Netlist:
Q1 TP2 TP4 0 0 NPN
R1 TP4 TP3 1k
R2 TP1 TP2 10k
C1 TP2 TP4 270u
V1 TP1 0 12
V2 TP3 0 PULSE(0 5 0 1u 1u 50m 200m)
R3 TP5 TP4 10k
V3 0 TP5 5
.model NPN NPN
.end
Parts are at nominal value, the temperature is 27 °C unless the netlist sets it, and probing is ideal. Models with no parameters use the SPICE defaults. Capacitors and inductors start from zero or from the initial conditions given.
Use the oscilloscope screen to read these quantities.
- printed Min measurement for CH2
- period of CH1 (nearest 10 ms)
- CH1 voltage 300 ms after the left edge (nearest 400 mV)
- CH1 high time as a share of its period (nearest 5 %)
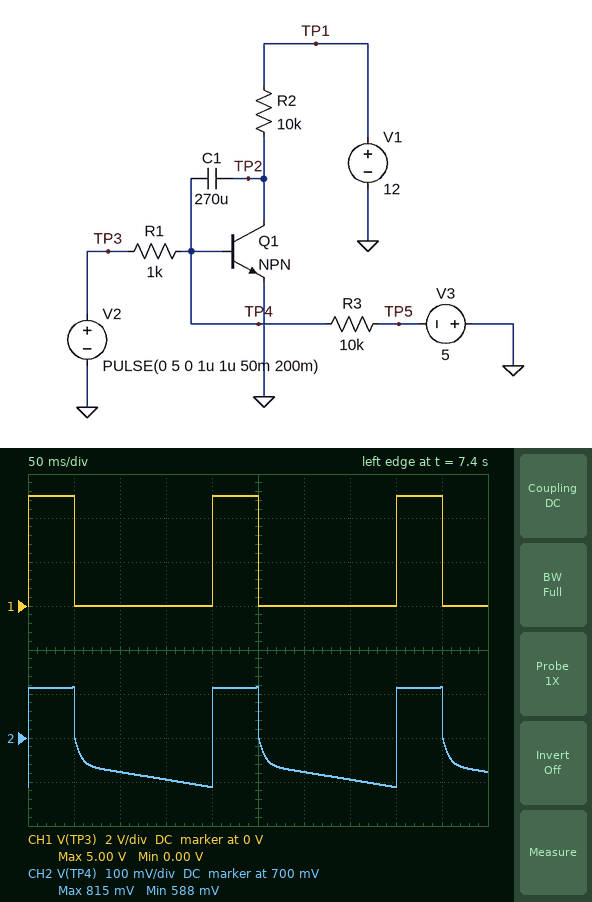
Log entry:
588 mV
200 ms
0 V
25 %
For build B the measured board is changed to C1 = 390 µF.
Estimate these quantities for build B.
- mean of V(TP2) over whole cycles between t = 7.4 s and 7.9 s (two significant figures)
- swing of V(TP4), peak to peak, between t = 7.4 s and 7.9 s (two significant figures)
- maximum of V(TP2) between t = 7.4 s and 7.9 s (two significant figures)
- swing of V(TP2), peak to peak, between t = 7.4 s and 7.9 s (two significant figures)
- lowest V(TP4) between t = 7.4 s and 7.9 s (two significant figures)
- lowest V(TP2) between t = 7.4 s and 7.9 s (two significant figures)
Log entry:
240 mV
220 mV
620 mV
630 mV
600 mV
-16 mV
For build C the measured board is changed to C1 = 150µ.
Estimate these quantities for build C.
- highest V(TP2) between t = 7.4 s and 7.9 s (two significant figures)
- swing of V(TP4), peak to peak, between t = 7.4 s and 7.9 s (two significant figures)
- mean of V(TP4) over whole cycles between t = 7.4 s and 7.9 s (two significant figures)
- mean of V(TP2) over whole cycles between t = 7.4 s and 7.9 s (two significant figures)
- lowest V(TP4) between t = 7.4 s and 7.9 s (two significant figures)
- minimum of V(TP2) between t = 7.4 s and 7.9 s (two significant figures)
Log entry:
1.2 V
270 mV
650 mV
480 mV
550 mV
-28 mV
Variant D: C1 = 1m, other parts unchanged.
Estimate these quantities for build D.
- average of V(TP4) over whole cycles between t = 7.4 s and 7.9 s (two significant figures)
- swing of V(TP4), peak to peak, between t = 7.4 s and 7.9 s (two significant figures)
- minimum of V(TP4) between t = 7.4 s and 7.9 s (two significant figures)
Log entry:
660 mV
220 mV
600 mV
